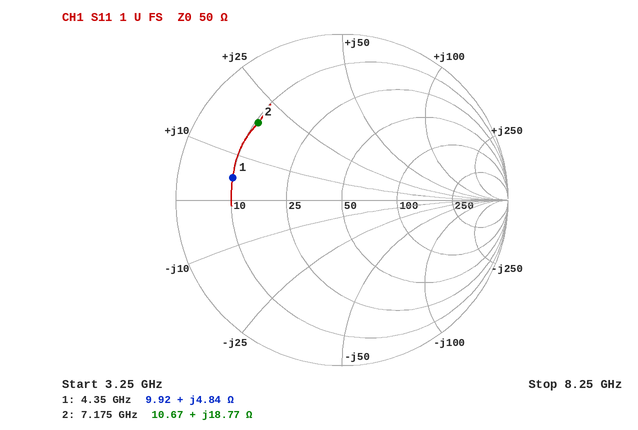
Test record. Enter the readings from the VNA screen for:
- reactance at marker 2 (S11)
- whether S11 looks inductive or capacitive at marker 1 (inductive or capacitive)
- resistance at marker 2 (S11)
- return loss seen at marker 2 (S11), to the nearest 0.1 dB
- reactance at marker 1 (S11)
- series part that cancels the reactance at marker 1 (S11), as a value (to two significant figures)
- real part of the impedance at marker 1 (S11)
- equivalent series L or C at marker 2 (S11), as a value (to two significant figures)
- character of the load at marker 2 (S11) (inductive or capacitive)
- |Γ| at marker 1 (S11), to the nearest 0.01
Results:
+18.77 Ω
inductive
10.67 Ω
3.3 dB
+4.84 Ω
7.6 pF
9.92 Ω
420 pH
inductive
0.67
